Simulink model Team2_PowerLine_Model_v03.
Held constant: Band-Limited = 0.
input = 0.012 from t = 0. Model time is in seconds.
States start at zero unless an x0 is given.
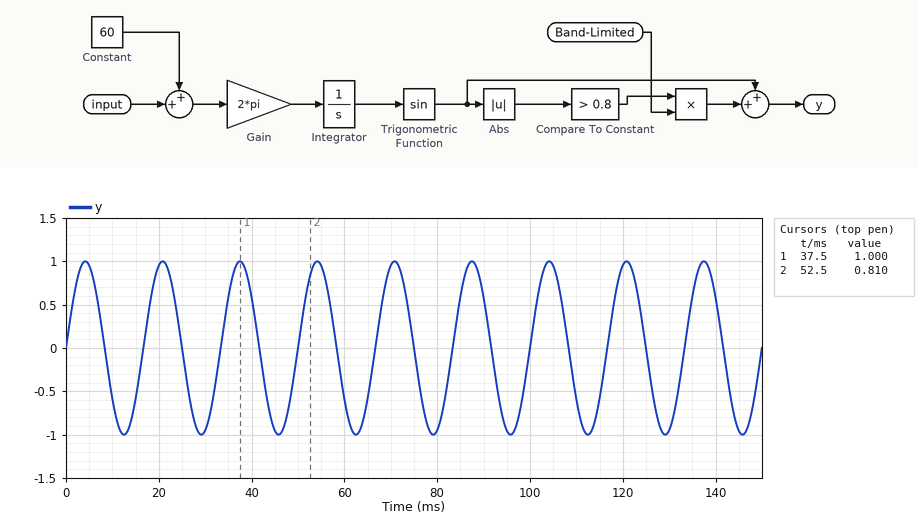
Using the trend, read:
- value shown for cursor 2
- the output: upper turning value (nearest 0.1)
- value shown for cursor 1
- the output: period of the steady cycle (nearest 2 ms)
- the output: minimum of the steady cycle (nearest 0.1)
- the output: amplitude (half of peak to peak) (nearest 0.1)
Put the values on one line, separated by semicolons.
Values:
0.810; 1.0; 1.000; 16 ms; -1.0; 1.0
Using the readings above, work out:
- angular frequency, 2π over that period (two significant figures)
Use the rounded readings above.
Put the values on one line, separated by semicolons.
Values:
0.39 rad/ms
